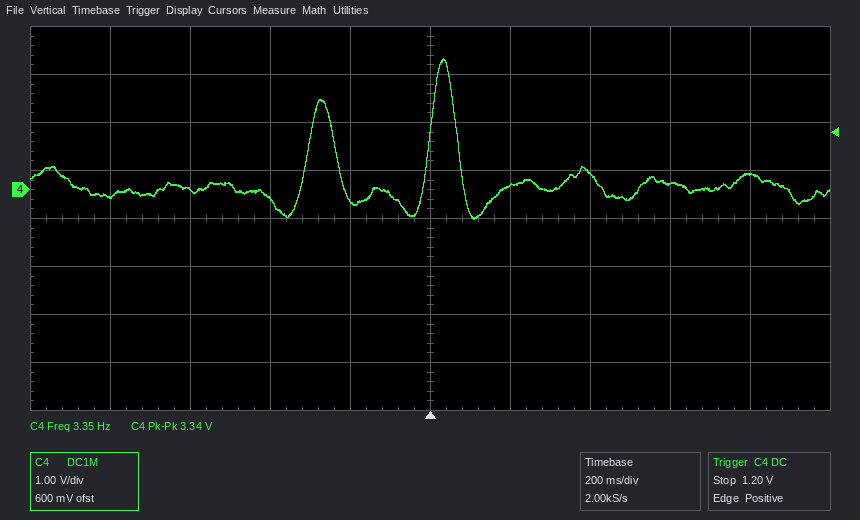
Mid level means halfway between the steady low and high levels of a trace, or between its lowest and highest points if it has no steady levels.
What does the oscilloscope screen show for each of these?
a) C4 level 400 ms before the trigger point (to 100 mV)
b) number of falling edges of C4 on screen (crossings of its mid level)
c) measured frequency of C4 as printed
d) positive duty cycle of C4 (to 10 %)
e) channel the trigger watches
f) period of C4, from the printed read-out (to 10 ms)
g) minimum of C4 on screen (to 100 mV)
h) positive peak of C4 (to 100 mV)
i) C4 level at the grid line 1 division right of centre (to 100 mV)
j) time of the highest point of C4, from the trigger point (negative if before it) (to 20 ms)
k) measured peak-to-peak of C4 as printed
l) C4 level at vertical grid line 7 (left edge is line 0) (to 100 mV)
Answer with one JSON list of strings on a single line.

["-200 mV", "2", "3.35 Hz", "20 %", "C4", "300 ms", "-600 mV", "2.7 V", "100 mV", "+40 ms", "3.34 V", "300 mV"]
